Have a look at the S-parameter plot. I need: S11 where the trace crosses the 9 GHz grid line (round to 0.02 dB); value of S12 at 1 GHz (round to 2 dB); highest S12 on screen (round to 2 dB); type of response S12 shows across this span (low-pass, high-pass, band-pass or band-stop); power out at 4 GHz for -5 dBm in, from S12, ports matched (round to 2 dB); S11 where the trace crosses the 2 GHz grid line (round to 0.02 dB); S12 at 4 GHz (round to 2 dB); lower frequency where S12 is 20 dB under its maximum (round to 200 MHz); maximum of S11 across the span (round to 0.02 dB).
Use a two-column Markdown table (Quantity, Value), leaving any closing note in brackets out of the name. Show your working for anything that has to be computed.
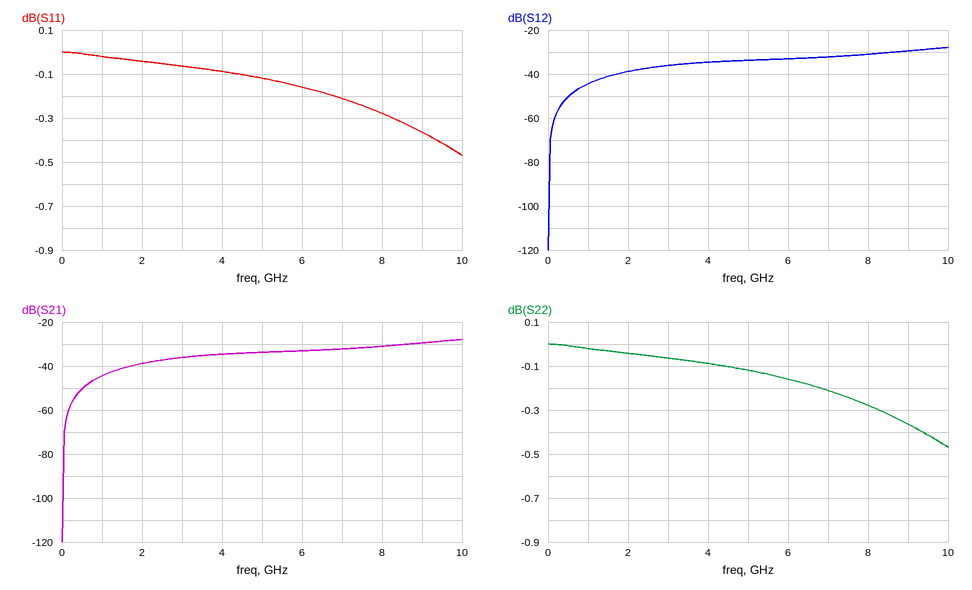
| Quantity | Value |
|---|---|
| S11 where the trace crosses the 9 GHz grid line | -0.36 dB |
| value of S12 at 1 GHz | -44 dB |
| highest S12 on screen | -28 dB |
| type of response S12 shows across this span | high-pass |
| power out at 4 GHz for -5 dBm in, from S12, ports matched | -5 dBm + (-34 dB) = -40 dBm |
| S11 where the trace crosses the 2 GHz grid line | -0.04 dB |
| S12 at 4 GHz | -34 dB |
| lower frequency where S12 is 20 dB under its maximum | 600 MHz |
| maximum of S11 across the span | 0.00 dB |
